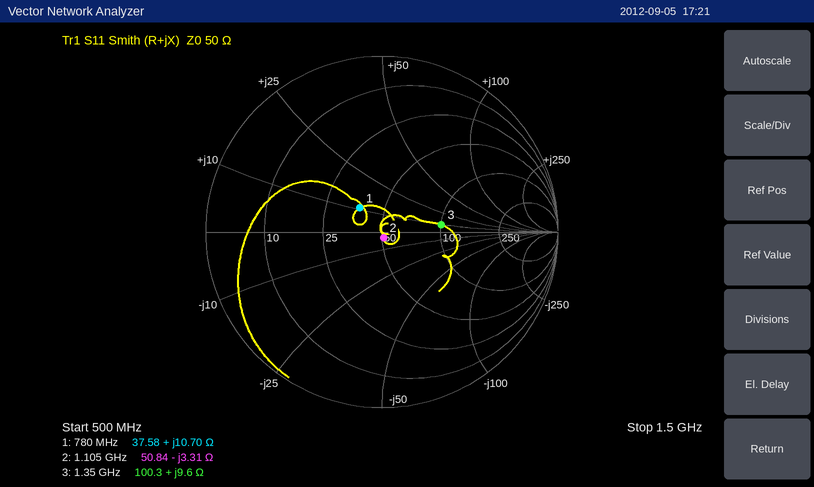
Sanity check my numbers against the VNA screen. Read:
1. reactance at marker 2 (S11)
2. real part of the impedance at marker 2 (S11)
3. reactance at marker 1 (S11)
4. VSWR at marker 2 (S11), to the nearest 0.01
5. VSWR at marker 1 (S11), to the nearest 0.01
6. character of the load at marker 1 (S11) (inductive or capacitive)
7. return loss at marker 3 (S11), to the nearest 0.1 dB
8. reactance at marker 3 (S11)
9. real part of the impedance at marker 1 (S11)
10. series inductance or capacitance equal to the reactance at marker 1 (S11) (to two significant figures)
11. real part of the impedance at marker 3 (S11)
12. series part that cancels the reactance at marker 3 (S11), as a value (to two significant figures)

-3.31 Ω
50.84 Ω
+10.70 Ω
1.07
1.46
inductive
9.4 dB
+9.6 Ω
37.58 Ω
2.2 nH
100.3 Ω
12 pF
